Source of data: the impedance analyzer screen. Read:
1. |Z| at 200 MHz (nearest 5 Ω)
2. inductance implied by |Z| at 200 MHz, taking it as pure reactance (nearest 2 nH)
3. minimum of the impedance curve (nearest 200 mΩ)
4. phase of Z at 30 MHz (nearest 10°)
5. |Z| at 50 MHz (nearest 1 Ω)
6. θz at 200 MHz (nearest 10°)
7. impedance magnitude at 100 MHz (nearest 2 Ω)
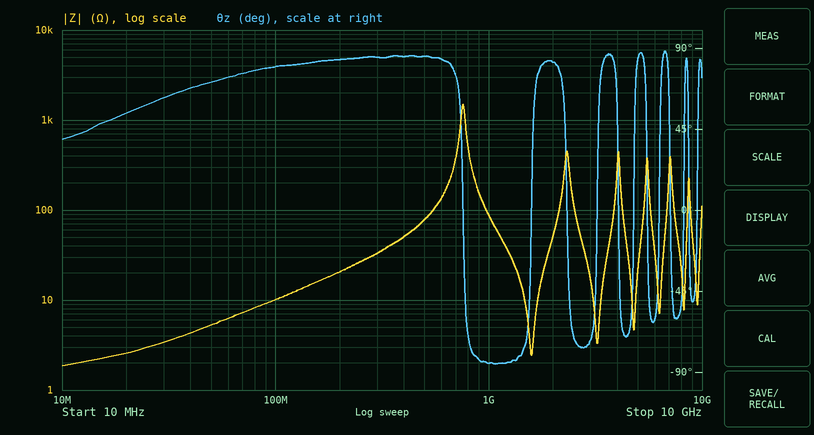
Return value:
20 Ω
16 nH
1.8 Ω
60°
5 Ω
80°
10 Ω
